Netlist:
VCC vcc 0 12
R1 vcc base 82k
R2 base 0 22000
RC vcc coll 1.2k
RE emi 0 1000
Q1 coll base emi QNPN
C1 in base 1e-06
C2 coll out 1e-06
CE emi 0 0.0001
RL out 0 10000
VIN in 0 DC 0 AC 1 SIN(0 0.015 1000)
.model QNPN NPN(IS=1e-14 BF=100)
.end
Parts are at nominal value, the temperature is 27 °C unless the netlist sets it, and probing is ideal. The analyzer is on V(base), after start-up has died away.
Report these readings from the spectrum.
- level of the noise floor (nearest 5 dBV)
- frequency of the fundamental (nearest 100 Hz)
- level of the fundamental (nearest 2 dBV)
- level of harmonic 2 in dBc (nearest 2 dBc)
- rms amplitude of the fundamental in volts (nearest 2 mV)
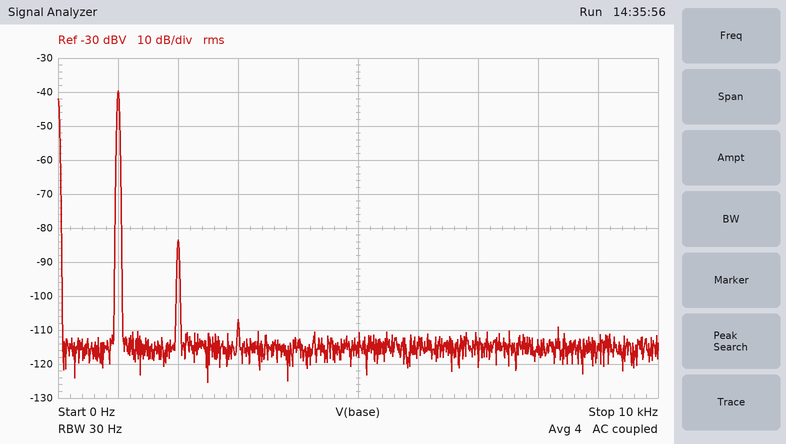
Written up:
-115 dBV
1.0 kHz
-40 dBV
-44 dBc
10 mV
